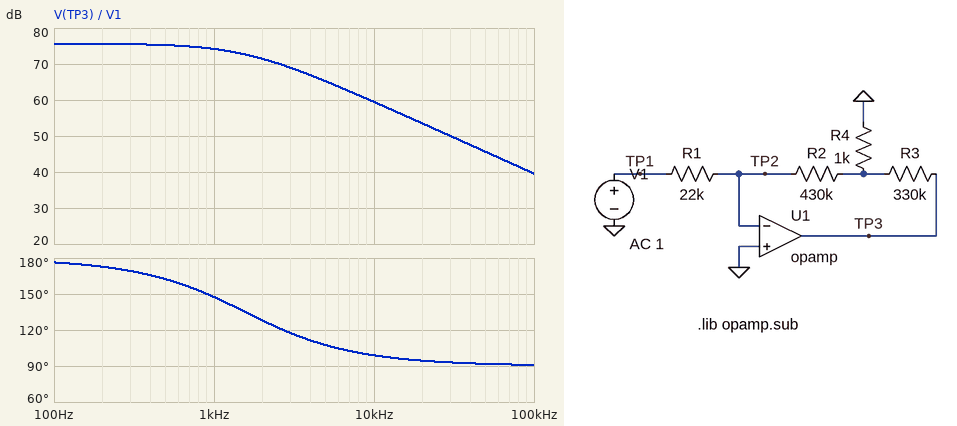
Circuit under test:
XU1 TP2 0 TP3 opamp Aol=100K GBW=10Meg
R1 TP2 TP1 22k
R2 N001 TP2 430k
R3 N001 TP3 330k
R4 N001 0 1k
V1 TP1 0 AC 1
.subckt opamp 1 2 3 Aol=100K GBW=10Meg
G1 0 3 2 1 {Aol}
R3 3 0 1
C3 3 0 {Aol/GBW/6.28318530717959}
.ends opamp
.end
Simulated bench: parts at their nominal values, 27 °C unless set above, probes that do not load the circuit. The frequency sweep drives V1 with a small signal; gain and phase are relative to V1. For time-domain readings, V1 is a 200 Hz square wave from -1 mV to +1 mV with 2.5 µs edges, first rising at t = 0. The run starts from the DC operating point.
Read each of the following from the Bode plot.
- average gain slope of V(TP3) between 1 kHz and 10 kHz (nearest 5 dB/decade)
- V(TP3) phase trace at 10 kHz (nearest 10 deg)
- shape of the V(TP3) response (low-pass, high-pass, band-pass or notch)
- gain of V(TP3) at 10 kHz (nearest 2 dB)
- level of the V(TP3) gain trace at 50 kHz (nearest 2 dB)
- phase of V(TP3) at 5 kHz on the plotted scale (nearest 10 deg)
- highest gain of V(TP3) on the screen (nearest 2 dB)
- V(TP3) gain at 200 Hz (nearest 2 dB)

-15 dB/decade
100 deg
low-pass
60 dB
46 dB
110 deg
76 dB
76 dB
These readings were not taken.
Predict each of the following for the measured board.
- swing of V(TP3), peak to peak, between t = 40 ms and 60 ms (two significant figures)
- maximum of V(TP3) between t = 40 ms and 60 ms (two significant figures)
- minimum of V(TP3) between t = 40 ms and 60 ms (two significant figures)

12 V
6.1 V
-6.1 V
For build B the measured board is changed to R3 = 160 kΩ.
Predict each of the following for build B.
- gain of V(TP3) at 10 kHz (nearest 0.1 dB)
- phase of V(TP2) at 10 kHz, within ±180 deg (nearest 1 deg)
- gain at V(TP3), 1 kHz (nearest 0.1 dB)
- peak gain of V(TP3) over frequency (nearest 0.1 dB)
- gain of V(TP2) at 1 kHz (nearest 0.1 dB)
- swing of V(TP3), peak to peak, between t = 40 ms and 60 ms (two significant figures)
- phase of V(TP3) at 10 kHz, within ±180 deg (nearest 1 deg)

59.2 dB
17 deg
69.3 dB
69.7 dB
-10.7 dB
6.1 V
107 deg
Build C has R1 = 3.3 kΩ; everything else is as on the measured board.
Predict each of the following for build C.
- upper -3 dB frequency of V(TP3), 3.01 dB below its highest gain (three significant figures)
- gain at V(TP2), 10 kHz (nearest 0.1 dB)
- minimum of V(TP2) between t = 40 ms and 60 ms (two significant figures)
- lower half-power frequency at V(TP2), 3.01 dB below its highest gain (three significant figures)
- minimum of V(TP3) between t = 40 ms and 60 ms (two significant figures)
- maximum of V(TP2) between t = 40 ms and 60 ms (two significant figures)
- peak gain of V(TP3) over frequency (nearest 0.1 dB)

330 Hz
-0.1 dB
-1.7 mV
298 Hz
-30 V
1.7 mV
89.6 dB
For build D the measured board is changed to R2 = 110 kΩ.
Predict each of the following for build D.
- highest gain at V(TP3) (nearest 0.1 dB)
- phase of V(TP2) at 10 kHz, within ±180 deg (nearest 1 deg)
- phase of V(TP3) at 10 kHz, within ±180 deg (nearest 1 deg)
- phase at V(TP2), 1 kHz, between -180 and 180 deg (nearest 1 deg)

64.3 dB
26 deg
117 deg
73 deg
